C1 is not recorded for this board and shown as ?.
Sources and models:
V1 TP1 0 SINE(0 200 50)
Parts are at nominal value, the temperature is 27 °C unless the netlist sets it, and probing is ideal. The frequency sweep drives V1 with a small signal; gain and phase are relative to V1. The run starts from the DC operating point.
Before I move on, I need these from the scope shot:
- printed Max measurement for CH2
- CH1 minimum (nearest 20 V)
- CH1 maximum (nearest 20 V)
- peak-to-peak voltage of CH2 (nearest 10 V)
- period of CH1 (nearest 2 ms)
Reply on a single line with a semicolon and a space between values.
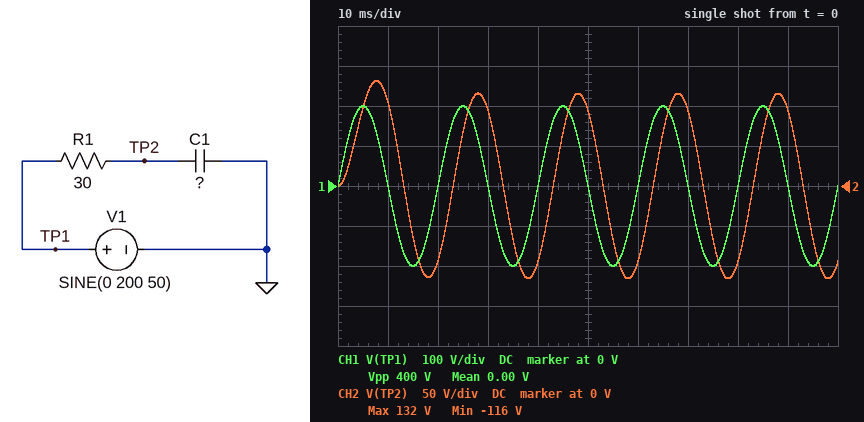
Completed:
132 V; -200 V; 200 V; 250 V; 20 ms
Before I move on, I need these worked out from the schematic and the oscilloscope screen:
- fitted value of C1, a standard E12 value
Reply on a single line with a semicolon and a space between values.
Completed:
150 µF
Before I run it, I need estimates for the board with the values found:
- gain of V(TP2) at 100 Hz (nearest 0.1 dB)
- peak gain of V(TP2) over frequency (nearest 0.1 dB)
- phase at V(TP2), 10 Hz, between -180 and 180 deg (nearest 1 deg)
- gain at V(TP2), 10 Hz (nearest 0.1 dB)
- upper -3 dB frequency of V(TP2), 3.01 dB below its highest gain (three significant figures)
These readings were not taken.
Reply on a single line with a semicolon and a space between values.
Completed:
-9.5 dB; 0 dB; -16 deg; -0.3 dB; 35.4 Hz
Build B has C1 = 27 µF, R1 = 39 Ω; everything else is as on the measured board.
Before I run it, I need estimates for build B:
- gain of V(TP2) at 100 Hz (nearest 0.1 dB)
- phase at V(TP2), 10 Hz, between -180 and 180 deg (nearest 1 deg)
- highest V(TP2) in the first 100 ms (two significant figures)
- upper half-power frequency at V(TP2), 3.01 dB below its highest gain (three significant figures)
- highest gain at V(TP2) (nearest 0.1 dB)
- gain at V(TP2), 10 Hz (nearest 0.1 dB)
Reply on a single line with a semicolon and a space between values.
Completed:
-1.6 dB; -4 deg; 190 V; 151 Hz; 0 dB; 0 dB
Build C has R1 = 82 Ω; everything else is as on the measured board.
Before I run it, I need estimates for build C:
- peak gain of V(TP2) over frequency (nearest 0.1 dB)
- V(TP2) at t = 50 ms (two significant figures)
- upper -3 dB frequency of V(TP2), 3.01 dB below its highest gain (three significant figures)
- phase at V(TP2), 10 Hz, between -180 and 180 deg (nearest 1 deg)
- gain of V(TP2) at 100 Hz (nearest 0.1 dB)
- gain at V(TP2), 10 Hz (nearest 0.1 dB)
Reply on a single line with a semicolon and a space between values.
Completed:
0 dB; 49 V; 12.9 Hz; -38 deg; -17.8 dB; -2.0 dB
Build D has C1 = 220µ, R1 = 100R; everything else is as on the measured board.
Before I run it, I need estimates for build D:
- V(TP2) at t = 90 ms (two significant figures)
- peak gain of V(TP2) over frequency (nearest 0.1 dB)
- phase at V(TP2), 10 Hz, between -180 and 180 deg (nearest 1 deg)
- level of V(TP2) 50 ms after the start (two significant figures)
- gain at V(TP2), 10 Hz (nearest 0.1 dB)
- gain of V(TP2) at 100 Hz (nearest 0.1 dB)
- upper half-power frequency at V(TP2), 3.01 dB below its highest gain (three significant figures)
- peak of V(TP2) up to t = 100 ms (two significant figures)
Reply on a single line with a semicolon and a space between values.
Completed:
29 V; 0 dB; -54 deg; 31 V; -4.6 dB; -22.8 dB; 7.23 Hz; 47 V
